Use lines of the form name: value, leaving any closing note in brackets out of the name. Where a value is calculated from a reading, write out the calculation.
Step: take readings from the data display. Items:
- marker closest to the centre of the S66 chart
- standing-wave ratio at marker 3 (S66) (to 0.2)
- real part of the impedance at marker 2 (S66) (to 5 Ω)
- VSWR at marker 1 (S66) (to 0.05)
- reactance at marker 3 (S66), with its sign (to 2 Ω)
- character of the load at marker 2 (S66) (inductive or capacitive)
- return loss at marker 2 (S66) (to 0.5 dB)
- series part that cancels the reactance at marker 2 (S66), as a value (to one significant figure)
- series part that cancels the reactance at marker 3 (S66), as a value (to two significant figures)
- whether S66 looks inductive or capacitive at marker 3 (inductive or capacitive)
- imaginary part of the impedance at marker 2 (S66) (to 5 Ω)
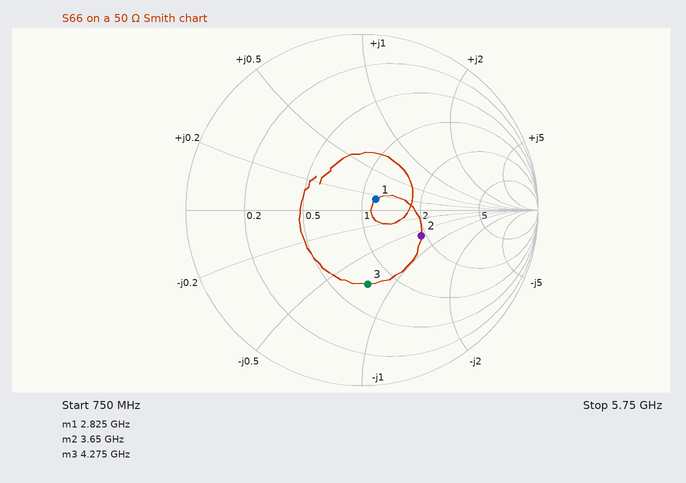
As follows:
marker closest to the centre of the S66 chart: marker 1
standing-wave ratio at marker 3 (S66): 2.4
real part of the impedance at marker 2 (S66): 95 Ω
VSWR at marker 1 (S66): 1.20
reactance at marker 3 (S66), with its sign: -38 Ω
character of the load at marker 2 (S66): capacitive
return loss at marker 2 (S66): 8.5 dB
series part that cancels the reactance at marker 2 (S66), as a value: L = 30 Ω/(2π × 3.65 GHz) ≈ 1 nH
series part that cancels the reactance at marker 3 (S66), as a value: L = 38 Ω/(2π × 4.275 GHz) ≈ 1.4 nH
whether S66 looks inductive or capacitive at marker 3: capacitive
imaginary part of the impedance at marker 2 (S66): -30 Ω
